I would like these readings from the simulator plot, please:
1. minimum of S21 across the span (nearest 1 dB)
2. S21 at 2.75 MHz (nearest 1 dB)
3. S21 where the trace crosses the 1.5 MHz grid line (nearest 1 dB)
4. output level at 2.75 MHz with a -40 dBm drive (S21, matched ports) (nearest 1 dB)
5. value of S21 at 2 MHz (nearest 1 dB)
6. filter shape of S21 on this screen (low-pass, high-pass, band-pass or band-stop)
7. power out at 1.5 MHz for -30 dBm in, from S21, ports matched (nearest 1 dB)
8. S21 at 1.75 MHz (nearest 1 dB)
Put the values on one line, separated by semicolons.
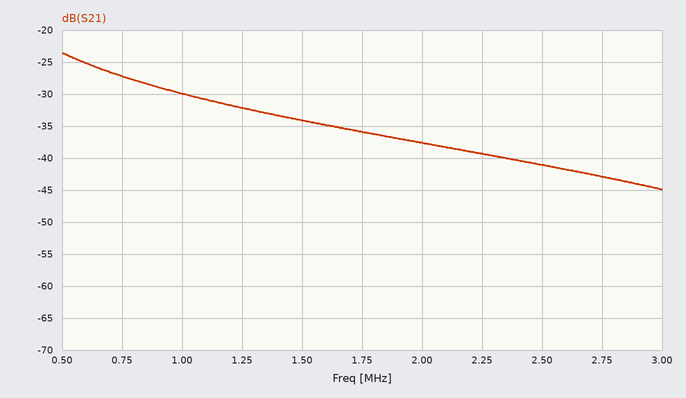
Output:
-45 dB; -43 dB; -34 dB; -83 dBm; -38 dB; low-pass; -64 dBm; -36 dB
